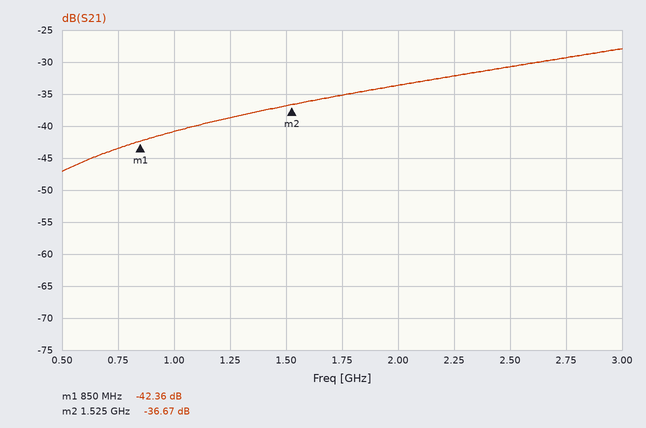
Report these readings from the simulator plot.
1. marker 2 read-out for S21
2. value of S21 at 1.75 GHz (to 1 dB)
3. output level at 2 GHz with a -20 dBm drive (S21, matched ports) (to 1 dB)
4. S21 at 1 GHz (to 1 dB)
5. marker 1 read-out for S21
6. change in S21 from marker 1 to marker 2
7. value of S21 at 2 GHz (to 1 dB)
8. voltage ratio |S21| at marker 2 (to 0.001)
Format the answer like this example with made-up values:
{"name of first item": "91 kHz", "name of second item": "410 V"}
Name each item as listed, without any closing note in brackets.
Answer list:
{"marker 2 read-out for S21": "-36.67 dB", "value of S21 at 1.75 GHz": "-35 dB", "output level at 2 GHz with a -20 dBm drive (S21, matched ports)": "-54 dBm", "S21 at 1 GHz": "-41 dB", "marker 1 read-out for S21": "-42.36 dB", "change in S21 from marker 1 to marker 2": "5.69 dB", "value of S21 at 2 GHz": "-34 dB", "voltage ratio |S21| at marker 2": "0.015"}
